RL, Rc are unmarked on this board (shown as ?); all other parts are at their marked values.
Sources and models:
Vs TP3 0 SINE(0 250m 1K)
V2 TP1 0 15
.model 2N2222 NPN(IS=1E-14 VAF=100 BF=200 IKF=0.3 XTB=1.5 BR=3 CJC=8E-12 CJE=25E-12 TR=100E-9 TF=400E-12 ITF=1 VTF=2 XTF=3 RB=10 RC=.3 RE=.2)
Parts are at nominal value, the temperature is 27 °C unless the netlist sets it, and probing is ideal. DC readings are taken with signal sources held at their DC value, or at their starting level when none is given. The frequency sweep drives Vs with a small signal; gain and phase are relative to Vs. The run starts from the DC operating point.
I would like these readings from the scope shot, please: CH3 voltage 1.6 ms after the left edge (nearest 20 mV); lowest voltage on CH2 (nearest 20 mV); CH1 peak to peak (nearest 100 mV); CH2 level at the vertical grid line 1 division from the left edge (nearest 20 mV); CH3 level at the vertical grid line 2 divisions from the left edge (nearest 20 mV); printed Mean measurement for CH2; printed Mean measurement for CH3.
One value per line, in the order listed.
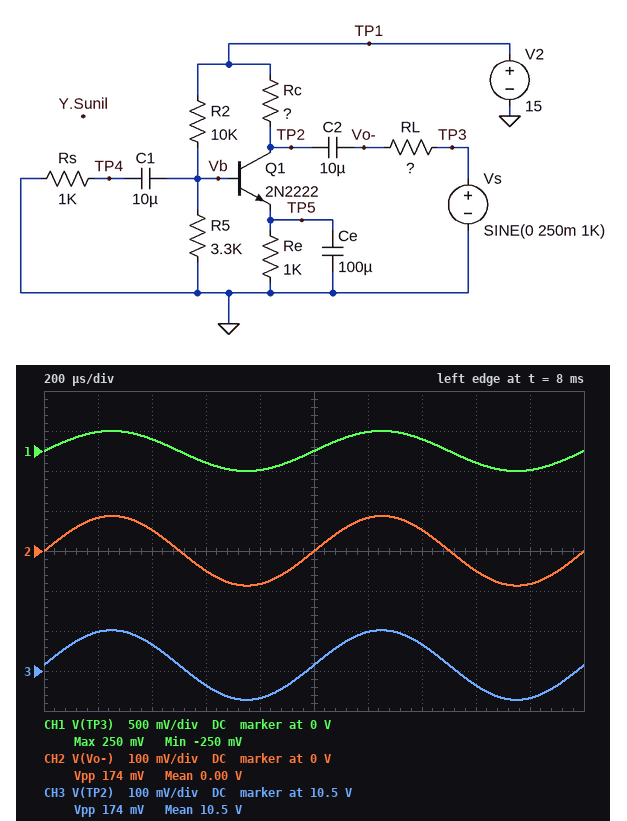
10.46 V
-80 mV
500 mV
80 mV
10.56 V
0.00 V
10.5 V
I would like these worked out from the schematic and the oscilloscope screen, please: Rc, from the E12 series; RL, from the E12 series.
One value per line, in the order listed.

1.5 kΩ
2.7 kΩ
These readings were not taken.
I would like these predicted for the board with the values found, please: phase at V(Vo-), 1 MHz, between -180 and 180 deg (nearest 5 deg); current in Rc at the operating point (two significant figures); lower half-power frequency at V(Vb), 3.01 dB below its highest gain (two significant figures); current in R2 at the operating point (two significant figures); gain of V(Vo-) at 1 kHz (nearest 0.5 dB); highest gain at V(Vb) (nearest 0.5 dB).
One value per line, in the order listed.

-40 deg
3.0 mA
630 kHz
1.1 mA
-9.0 dB
-51.5 dB
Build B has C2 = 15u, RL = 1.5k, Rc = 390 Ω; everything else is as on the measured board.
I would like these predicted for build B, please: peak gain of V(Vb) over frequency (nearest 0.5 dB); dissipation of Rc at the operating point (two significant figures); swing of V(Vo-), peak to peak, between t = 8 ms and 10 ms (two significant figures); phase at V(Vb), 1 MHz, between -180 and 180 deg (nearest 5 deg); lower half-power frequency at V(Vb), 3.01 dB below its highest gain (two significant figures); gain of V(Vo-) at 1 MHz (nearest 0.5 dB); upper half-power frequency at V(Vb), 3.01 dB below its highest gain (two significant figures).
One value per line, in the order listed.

-49.5 dB
3.5 mW
100 mV
55 deg
1.5 MHz
-15.0 dB
380 MHz
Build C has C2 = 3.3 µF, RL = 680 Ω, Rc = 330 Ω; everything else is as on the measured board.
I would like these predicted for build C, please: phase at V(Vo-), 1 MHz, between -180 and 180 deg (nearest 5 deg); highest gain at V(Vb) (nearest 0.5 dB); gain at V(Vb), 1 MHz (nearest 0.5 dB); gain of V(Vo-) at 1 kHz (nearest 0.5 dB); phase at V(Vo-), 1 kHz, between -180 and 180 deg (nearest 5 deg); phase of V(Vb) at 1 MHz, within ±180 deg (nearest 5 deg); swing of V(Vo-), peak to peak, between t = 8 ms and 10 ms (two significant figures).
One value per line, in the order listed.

-15 deg
-44.0 dB
-50.5 dB
-9.5 dB
-5 deg
60 deg
160 mV
